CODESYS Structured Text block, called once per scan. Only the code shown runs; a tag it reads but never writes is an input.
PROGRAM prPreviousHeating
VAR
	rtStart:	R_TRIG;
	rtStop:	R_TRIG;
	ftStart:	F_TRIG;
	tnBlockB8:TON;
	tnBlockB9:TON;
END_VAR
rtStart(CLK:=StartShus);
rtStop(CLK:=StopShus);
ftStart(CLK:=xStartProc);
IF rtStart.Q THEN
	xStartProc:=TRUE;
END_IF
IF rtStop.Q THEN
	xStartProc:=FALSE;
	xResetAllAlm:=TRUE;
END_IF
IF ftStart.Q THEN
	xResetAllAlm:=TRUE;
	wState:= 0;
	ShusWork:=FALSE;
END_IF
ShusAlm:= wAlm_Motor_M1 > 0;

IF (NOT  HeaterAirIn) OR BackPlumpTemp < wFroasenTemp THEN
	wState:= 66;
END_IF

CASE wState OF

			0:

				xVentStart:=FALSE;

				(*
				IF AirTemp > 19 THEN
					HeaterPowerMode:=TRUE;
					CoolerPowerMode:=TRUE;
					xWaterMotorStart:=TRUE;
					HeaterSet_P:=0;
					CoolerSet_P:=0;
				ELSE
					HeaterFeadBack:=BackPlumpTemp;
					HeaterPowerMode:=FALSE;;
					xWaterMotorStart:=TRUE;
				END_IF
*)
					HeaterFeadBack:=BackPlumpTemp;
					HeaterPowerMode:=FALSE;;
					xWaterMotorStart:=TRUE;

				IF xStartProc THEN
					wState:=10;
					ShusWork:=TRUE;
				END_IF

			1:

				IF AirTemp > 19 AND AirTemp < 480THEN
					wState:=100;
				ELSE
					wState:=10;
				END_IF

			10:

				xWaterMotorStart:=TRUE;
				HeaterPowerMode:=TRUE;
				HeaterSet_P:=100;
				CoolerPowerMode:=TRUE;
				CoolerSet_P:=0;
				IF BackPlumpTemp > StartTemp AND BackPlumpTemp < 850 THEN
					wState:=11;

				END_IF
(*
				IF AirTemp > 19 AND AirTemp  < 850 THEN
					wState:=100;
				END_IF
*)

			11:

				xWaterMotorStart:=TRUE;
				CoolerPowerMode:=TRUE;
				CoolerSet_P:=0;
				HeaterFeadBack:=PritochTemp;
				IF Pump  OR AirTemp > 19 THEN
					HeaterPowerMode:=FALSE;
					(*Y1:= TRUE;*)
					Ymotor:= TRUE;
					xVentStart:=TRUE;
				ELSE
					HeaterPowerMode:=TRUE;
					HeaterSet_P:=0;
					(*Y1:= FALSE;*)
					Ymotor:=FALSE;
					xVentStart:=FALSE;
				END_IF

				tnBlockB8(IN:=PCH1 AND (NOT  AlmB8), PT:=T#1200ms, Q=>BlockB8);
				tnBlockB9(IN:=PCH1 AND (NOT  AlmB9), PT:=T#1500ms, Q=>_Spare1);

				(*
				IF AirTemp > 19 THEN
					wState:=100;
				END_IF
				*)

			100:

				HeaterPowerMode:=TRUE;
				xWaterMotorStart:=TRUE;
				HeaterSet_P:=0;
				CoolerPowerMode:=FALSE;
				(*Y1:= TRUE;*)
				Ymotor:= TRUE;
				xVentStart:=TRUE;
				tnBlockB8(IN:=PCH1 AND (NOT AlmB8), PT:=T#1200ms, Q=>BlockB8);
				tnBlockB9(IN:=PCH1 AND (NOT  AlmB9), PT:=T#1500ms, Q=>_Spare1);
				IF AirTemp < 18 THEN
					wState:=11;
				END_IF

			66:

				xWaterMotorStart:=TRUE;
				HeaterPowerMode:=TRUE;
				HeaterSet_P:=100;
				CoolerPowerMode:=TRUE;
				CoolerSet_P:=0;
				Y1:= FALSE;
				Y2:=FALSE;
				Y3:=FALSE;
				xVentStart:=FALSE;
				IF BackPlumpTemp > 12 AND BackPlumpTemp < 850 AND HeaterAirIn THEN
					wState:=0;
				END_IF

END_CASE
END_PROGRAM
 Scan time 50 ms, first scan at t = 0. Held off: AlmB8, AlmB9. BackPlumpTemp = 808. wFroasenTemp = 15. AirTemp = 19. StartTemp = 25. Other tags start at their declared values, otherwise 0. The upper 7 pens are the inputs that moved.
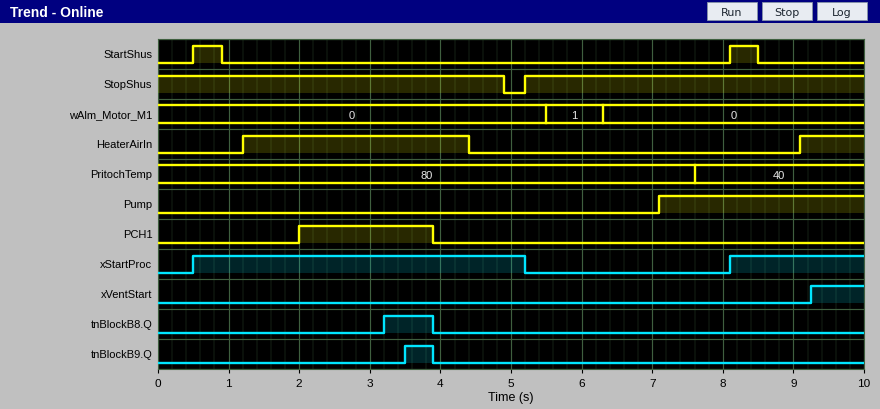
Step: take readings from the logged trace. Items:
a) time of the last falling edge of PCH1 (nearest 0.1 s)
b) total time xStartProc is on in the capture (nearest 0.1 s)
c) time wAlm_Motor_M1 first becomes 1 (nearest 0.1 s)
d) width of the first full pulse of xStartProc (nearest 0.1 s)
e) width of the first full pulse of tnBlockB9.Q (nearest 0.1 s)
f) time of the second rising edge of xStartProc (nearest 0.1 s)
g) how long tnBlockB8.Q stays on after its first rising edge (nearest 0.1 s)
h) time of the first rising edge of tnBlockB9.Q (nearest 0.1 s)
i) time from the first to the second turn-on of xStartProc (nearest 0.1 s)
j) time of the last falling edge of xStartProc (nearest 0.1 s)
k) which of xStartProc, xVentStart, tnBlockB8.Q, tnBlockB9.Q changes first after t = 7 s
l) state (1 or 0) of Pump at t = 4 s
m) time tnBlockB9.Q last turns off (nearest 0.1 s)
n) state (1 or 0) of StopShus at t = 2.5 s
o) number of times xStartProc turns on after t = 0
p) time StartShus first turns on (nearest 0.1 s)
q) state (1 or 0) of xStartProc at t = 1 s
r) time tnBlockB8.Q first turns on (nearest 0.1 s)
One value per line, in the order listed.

3.9 s
6.6 s
5.5 s
4.7 s
0.4 s
8.1 s
0.7 s
3.5 s
7.6 s
5.2 s
xStartProc
0
3.9 s
1
2
0.5 s
1
3.2 s
